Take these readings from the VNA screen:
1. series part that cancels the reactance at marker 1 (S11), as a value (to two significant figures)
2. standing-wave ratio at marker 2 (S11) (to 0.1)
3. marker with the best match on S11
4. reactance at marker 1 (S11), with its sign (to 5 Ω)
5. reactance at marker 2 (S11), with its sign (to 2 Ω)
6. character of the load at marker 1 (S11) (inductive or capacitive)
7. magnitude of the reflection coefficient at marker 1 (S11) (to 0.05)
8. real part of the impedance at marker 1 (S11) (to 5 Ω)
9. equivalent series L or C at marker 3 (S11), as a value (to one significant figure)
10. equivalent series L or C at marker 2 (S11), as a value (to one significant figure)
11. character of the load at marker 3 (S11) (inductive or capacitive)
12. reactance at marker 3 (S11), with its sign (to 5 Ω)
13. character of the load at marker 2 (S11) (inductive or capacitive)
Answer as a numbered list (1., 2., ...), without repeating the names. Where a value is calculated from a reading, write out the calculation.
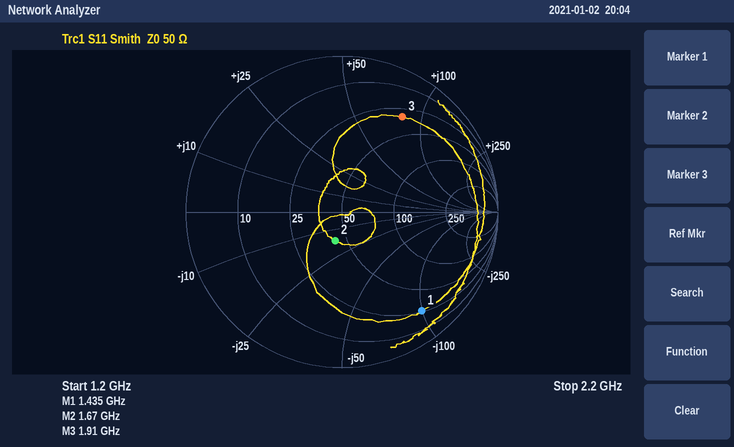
1. L = 100 Ω/(2π × 1.435 GHz) ≈ 11 nH
2. 1.5
3. marker 2
4. -100 Ω
5. -16 Ω
6. capacitive
7. 0.80
8. 25 Ω
9. L = 80 Ω/(2π × 1.91 GHz) ≈ 7 nH
10. C = 1/(2π × 1.67 GHz × 16 Ω) ≈ 6 pF
11. inductive
12. +80 Ω
13. capacitive
